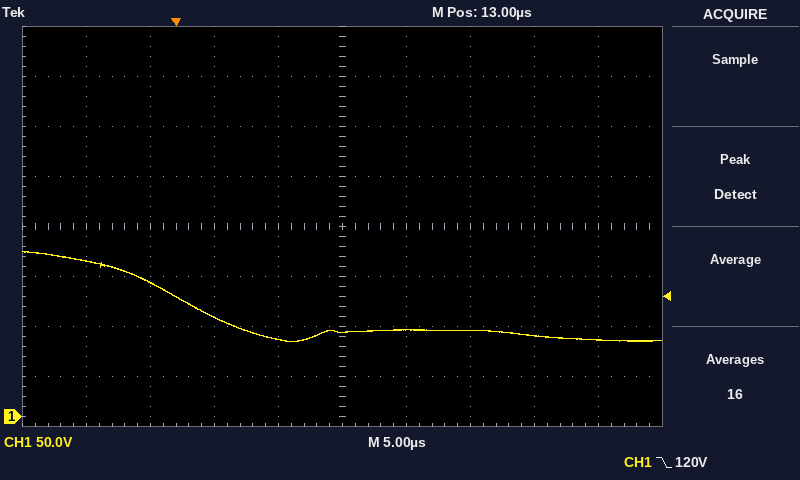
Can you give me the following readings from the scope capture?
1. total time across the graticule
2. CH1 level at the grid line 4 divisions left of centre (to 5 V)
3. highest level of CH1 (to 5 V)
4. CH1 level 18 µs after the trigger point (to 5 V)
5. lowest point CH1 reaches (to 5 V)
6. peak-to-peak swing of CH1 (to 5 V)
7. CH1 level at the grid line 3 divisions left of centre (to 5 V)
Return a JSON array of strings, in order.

["50 µs", "155 V", "165 V", "85 V", "75 V", "90 V", "135 V"]
